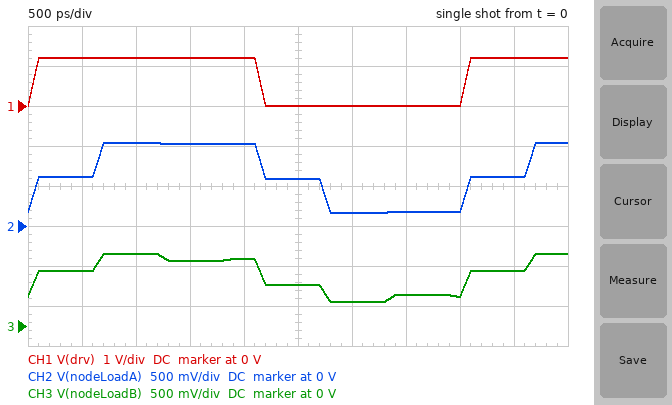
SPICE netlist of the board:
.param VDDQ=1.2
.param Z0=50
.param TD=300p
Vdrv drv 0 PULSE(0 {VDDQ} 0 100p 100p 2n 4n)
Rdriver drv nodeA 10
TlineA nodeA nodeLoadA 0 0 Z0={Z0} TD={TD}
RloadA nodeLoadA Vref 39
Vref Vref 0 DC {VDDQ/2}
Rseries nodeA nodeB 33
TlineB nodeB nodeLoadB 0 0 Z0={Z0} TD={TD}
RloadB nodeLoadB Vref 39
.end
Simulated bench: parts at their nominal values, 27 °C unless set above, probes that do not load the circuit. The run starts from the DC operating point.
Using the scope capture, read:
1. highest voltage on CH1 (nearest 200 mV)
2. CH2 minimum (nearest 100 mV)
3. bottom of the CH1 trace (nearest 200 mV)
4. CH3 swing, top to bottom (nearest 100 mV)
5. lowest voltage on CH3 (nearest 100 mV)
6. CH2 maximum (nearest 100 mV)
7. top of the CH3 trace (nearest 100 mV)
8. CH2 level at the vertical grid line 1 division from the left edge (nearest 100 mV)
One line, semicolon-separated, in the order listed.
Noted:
1.2 V; 200 mV; 0 V; 600 mV; 300 mV; 1.0 V; 900 mV; 600 mV
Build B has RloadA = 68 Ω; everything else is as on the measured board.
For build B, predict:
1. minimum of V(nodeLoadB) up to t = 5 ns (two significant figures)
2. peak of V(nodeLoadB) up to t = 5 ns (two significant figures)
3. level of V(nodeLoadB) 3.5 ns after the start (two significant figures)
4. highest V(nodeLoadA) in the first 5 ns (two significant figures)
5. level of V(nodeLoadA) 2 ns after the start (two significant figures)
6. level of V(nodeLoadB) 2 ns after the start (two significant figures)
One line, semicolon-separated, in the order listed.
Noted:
290 mV; 910 mV; 360 mV; 1.2 V; 1.1 V; 860 mV
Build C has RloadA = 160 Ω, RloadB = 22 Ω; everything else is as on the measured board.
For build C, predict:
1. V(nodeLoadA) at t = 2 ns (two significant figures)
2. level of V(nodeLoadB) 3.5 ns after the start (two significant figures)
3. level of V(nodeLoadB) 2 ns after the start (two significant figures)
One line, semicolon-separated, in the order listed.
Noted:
1.1 V; 410 mV; 790 mV
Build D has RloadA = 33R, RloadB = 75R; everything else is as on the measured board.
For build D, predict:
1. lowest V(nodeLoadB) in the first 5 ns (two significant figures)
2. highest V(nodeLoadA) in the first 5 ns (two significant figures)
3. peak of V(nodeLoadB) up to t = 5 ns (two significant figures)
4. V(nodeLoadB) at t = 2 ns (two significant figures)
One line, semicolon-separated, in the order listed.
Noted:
180 mV; 1.0 V; 1.0 V; 920 mV
